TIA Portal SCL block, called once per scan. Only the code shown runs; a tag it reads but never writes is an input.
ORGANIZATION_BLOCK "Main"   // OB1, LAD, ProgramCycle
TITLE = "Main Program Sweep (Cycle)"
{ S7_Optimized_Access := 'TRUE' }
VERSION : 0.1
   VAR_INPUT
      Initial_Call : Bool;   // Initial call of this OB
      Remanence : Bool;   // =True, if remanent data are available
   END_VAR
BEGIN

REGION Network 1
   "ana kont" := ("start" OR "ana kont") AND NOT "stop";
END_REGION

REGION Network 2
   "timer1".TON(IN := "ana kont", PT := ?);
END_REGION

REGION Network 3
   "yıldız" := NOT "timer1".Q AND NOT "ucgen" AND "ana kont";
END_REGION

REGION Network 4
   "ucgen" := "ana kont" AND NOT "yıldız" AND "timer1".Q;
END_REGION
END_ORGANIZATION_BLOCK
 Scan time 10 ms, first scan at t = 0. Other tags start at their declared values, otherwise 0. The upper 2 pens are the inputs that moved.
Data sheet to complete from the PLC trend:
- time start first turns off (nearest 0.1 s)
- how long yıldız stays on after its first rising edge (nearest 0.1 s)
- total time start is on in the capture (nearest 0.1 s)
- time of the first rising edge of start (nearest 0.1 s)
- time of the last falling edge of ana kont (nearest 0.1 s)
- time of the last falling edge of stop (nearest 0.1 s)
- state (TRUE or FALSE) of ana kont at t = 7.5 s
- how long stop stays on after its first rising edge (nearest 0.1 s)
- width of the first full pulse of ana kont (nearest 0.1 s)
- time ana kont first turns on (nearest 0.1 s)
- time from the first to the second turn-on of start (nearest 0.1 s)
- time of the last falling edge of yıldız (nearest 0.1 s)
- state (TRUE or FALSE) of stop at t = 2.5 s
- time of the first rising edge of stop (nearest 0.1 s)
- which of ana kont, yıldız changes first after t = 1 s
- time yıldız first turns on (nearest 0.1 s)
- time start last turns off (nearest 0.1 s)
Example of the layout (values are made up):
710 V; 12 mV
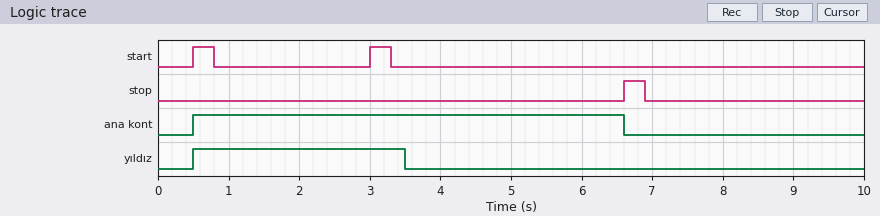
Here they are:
0.8 s; 3.0 s; 0.6 s; 0.5 s; 6.6 s; 6.9 s; FALSE; 0.3 s; 6.1 s; 0.5 s; 2.5 s; 3.5 s; FALSE; 6.6 s; yıldız; 0.5 s; 3.3 s
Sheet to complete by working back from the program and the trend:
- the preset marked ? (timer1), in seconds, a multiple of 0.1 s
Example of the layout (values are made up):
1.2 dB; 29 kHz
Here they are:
3.0 s
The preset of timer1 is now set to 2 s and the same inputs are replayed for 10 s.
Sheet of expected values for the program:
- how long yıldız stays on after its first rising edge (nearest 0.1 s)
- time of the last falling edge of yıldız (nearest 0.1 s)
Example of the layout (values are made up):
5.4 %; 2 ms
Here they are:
2.0 s; 2.5 s
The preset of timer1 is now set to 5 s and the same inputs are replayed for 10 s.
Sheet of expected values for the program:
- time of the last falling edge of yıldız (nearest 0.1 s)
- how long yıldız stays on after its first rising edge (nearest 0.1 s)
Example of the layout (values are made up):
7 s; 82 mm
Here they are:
5.5 s; 5.0 s
